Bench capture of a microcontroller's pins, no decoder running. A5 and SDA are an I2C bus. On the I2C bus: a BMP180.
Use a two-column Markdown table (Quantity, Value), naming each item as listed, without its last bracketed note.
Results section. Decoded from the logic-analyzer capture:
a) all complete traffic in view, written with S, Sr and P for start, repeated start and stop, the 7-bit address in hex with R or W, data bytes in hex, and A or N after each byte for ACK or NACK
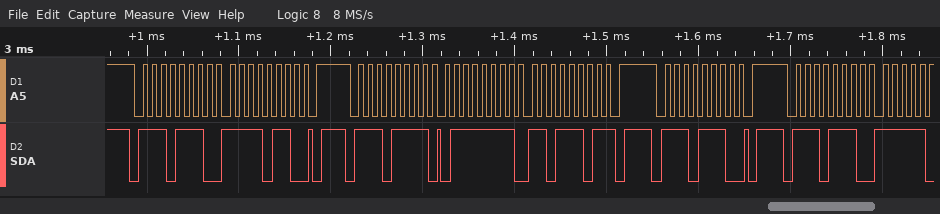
| Quantity | Value |
|---|---|
| all complete traffic in view, written with S, Sr and P for start, repeated start and stop, the 7-bit address in hex with R or W, data bytes in hex, and A or N after each byte for ACK or NACK | S 77W A F6 A P S 77R A 7F A DD N P S 77W A P S 77W A |
